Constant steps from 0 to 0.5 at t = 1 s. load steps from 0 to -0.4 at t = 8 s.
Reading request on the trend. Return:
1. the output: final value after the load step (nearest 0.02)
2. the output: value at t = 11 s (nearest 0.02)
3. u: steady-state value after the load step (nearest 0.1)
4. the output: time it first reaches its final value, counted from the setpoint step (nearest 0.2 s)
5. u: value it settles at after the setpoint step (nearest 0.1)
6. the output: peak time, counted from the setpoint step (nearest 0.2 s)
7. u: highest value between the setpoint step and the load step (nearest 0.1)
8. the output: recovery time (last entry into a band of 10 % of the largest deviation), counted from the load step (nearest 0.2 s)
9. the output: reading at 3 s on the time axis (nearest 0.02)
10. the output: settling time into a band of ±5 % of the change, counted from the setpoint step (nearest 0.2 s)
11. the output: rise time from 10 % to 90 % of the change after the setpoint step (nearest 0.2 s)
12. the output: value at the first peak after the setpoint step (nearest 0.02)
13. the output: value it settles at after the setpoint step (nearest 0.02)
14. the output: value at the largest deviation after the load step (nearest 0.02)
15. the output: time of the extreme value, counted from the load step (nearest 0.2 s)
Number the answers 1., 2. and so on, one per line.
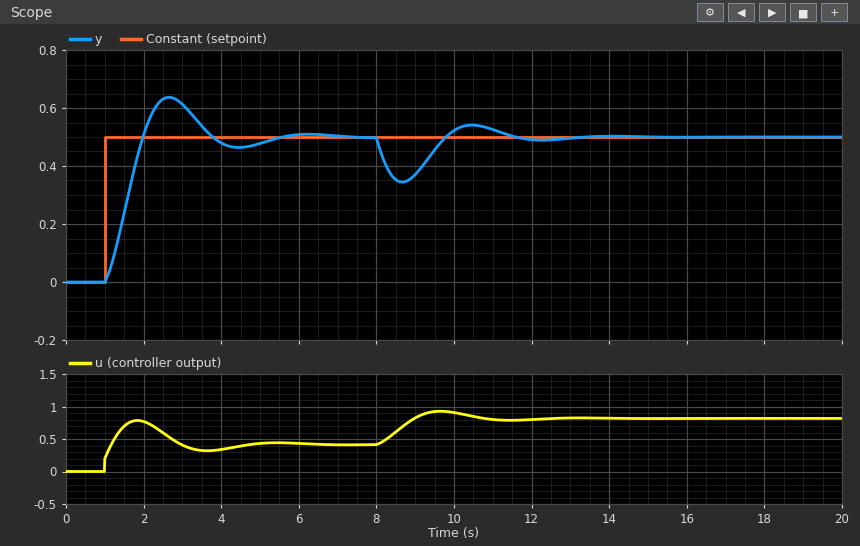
1. 0.50
2. 0.52
3. 0.8
4. 1.0 s
5. 0.4
6. 1.6 s
7. 0.8
8. 3.2 s
9. 0.62
10. 4.0 s
11. 0.8 s
12. 0.64
13. 0.50
14. 0.34
15. 0.6 s
